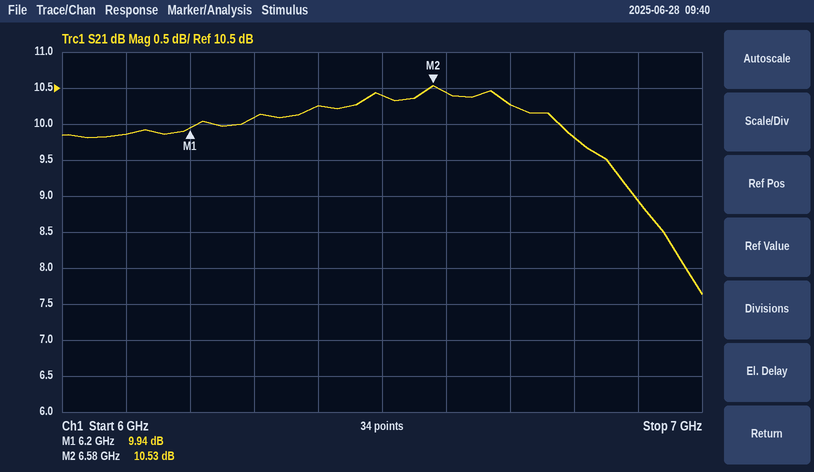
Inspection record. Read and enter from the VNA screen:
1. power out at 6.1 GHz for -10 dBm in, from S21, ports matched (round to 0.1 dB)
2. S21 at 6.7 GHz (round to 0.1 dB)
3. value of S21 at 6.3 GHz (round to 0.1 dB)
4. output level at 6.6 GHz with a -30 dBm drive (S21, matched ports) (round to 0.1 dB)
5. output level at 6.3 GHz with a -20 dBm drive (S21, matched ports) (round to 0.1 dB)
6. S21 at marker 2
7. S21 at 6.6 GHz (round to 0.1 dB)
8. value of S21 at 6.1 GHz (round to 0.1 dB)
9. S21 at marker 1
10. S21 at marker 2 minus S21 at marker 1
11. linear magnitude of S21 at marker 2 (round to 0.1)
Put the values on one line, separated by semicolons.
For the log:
-0.1 dBm; 10.3 dB; 10.1 dB; -19.6 dBm; -9.9 dBm; 10.53 dB; 10.4 dB; 9.9 dB; 9.94 dB; 0.59 dB; 3.4
